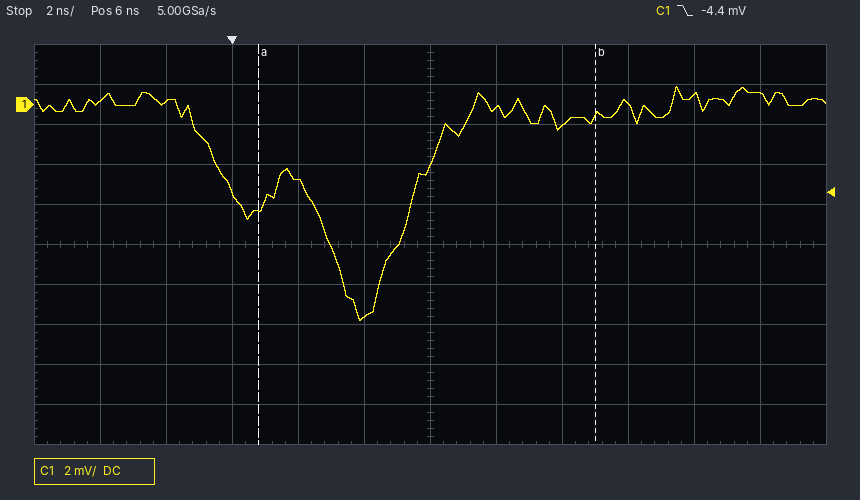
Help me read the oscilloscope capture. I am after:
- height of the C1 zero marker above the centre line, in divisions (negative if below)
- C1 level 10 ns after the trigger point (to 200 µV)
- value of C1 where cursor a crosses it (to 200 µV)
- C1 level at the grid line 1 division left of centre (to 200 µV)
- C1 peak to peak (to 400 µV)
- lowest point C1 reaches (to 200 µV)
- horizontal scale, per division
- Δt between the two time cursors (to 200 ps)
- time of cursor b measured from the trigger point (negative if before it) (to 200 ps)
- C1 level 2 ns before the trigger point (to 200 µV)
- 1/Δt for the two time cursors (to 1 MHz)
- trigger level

+3.5 div
-1.0 mV
-5.2 mV
-10.6 mV
11.6 mV
-10.8 mV
2 ns
10.2 ns
+11.0 ns
200 µV
98 MHz
-4.4 mV
